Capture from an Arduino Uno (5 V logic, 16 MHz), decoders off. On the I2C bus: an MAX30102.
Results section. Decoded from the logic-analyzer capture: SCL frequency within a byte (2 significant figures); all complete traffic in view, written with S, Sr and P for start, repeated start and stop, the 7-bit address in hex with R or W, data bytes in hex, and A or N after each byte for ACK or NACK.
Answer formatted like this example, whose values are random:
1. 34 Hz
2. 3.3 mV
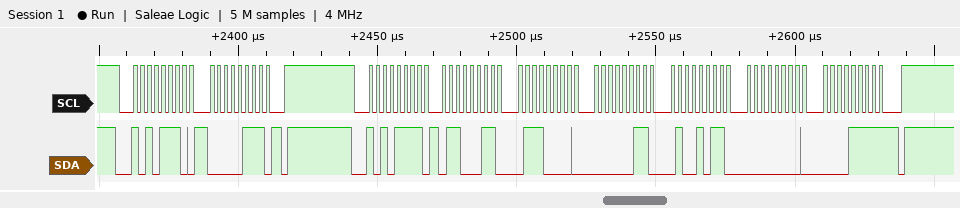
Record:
1. 400 kHz
2. S 57W A 07 A P S 57R A 63 A 70 A 03 A 4B A 00 A 0F N P
